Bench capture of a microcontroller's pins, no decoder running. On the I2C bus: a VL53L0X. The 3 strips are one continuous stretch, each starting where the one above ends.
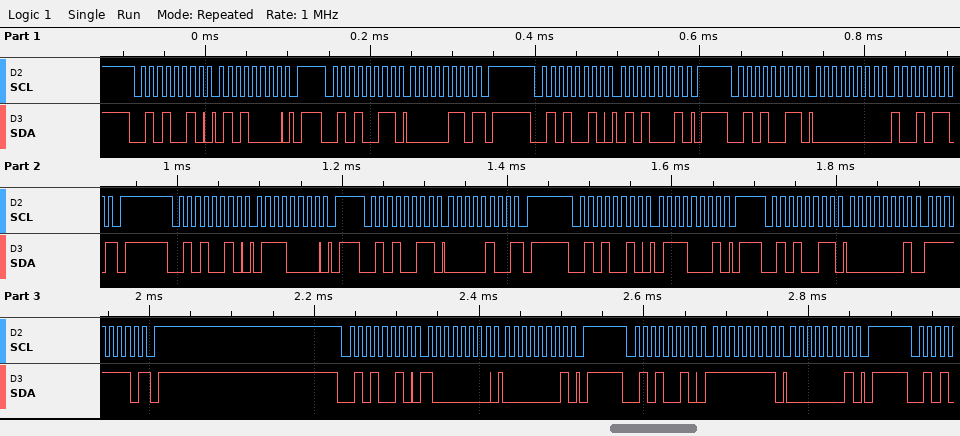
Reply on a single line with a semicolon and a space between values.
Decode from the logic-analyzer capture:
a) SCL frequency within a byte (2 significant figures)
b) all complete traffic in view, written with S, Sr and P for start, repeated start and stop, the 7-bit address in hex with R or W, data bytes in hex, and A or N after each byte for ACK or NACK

100 kHz; S 29W A 50 A P S 29R A 06 N P S 29W A 51 A P S 29R A 00 A 96 N P S 29W A 70 A P S 29R A 04 N P S 29W A 71 A P S 29R A 01 A FE N P S 29W A 80 A 01 A P S 29W A FF A 01 A P
